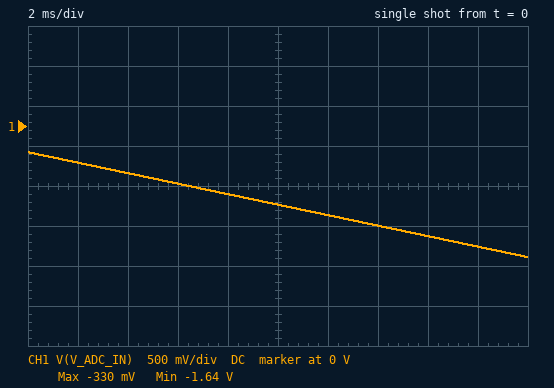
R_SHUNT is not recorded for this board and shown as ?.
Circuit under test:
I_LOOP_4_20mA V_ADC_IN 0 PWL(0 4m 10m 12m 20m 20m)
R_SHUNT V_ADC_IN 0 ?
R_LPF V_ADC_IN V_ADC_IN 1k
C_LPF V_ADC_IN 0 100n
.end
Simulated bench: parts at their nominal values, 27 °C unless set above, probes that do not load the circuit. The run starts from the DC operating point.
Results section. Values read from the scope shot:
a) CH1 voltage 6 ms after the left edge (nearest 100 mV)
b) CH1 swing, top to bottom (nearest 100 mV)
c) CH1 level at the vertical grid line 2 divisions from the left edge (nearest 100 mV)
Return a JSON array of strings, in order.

["-700 mV", "1.3 V", "-600 mV"]
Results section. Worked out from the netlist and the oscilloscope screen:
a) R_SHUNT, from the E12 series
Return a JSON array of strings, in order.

["82 Ω"]
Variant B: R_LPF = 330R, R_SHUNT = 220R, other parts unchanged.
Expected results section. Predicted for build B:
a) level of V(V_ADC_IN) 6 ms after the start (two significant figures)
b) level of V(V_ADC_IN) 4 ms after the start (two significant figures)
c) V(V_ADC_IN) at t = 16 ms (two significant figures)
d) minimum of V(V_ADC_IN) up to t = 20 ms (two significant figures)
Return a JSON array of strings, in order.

["-1.9 V", "-1.6 V", "-3.7 V", "-4.4 V"]
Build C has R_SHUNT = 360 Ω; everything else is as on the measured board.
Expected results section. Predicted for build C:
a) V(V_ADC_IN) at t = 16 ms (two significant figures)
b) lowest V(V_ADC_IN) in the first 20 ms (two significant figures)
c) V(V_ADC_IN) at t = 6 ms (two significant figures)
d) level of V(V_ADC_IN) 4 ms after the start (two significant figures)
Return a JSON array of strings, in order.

["-6.0 V", "-7.2 V", "-3.2 V", "-2.6 V"]
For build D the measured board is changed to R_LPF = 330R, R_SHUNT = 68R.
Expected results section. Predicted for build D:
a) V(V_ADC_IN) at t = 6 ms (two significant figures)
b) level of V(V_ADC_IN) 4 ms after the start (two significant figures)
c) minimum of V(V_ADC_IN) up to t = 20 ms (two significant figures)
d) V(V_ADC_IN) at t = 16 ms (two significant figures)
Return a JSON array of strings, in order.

["-600 mV", "-490 mV", "-1.4 V", "-1.1 V"]
